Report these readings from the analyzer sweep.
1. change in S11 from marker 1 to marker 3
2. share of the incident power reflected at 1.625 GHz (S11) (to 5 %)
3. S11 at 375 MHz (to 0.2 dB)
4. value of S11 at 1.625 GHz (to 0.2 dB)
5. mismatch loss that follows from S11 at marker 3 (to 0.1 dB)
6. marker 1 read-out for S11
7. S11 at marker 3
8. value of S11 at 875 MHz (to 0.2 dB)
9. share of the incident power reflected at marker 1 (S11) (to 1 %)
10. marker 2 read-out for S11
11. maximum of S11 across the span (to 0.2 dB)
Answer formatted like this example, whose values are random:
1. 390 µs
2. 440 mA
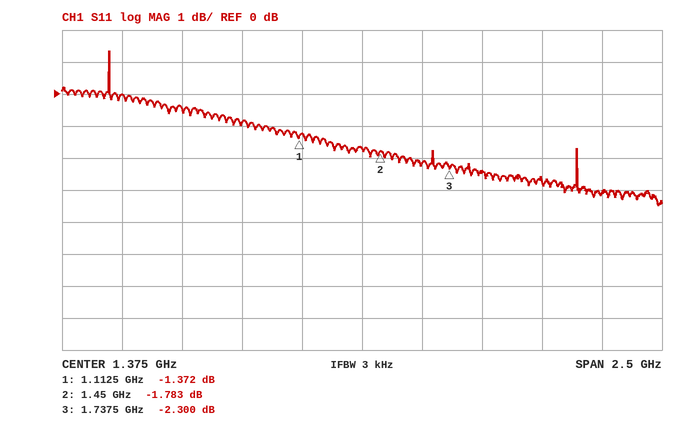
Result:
1. -0.928 dB
2. 60 %
3. 0.0 dB
4. -2.2 dB
5. 3.9 dB
6. -1.372 dB
7. -2.300 dB
8. -0.8 dB
9. 73 %
10. -1.783 dB
11. 1.4 dB
